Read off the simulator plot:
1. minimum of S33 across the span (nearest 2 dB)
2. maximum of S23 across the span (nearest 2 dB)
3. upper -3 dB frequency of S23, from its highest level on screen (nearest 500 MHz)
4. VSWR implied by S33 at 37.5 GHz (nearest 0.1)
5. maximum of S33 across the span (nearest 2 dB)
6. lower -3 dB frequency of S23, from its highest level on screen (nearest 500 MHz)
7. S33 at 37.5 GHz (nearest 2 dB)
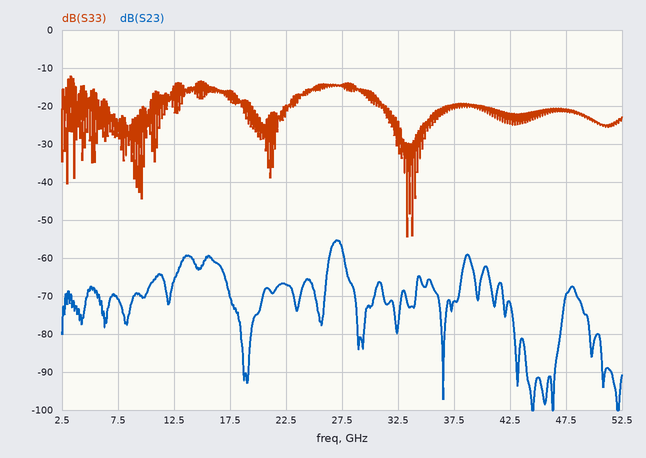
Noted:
-54 dB
-56 dB
27.5 GHz
1.2
-12 dB
26.5 GHz
-20 dB
